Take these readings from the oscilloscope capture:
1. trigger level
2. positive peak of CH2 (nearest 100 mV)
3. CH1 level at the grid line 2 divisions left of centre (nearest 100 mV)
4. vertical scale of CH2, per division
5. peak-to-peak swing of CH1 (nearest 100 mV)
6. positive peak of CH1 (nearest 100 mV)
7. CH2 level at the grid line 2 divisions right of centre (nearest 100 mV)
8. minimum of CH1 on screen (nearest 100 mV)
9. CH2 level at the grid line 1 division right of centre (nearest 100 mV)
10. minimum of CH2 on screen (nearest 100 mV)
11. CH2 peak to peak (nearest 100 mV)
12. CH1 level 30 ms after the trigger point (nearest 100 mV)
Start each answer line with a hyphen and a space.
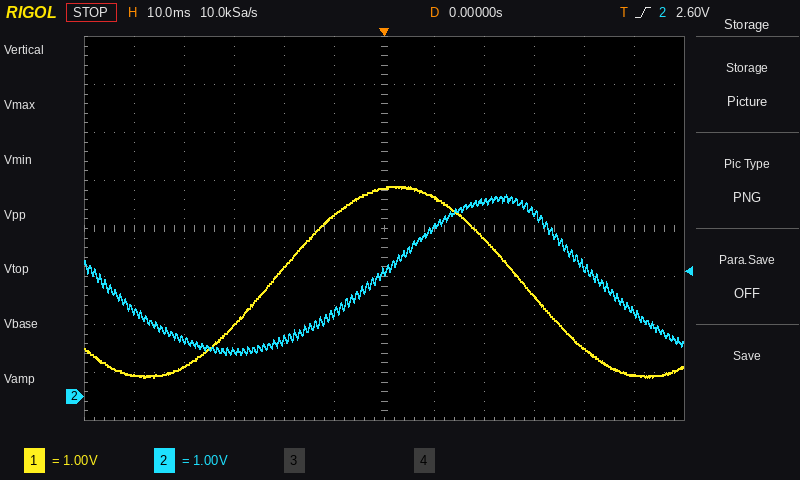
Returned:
- 2.60 V
- 4.2 V
- 2.7 V
- 1 V
- 4.0 V
- 4.4 V
- 4.1 V
- 400 mV
- 3.5 V
- 900 mV
- 3.3 V
- 2.1 V
